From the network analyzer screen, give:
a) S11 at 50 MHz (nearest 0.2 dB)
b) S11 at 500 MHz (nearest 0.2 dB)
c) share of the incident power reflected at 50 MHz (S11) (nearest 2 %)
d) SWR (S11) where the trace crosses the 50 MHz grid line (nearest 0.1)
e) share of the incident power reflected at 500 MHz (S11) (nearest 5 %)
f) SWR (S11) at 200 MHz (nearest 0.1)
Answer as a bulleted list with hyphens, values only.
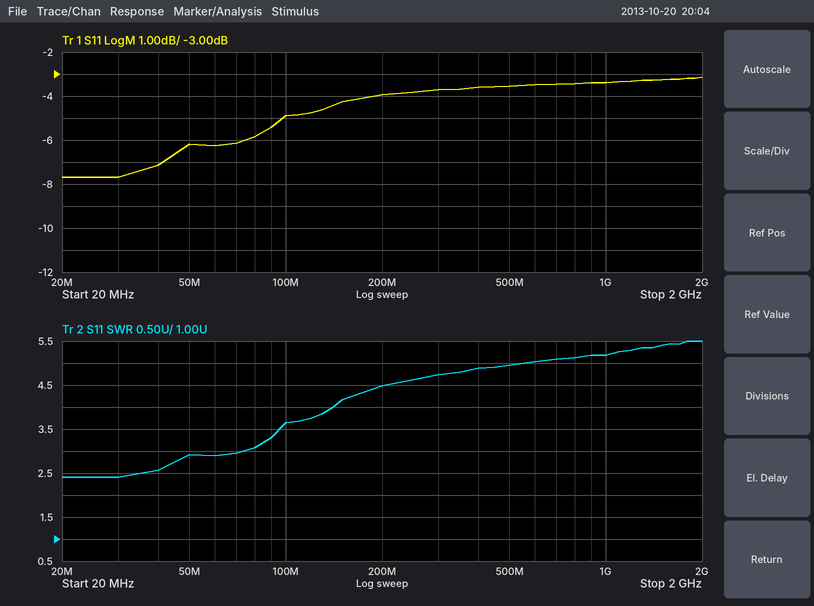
- -6.2 dB
- -3.6 dB
- 24 %
- 2.9
- 45 %
- 4.5
